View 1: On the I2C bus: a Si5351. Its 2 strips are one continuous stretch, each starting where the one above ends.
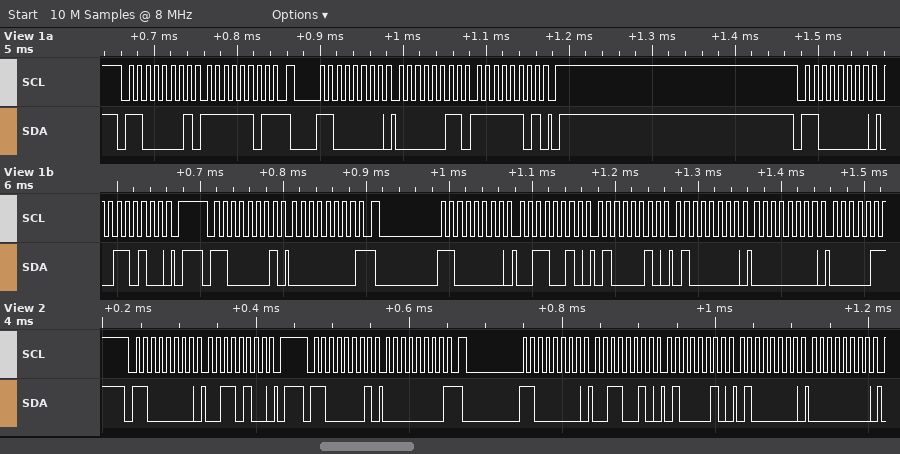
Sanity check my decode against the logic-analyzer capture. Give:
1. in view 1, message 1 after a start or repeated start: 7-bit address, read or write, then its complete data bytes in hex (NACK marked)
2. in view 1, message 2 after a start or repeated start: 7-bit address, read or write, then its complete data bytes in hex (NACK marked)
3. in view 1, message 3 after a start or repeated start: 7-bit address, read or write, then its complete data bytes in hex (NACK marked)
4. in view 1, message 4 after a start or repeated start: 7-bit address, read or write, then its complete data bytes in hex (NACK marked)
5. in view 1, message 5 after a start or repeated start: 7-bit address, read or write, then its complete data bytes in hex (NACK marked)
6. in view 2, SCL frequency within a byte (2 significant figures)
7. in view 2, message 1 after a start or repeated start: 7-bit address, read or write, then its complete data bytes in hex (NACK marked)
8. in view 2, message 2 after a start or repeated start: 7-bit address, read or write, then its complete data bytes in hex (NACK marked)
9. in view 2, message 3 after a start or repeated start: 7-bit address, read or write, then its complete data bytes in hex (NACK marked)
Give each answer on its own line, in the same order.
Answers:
0x60 read: FD NACK
0x60 write: 03 FD
0x60 write: 34
0x60 read: 00 NACK
0x60 write: 32 42 40 00
100 kHz
0x60 write: 34
0x60 read: 00 NACK
0x60 write: 32 42 40 00
